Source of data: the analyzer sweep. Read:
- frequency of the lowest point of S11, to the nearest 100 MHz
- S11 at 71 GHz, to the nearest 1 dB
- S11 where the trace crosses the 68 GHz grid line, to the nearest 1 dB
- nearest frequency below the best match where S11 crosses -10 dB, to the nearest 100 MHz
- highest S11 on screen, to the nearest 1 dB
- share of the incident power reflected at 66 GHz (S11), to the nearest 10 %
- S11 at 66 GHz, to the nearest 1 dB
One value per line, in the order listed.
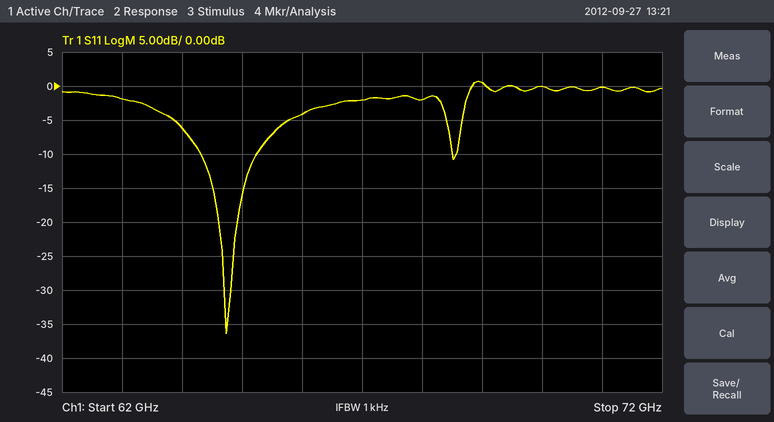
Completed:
64.7 GHz
0 dB
-2 dB
64.3 GHz
1 dB
40 %
-4 dB
